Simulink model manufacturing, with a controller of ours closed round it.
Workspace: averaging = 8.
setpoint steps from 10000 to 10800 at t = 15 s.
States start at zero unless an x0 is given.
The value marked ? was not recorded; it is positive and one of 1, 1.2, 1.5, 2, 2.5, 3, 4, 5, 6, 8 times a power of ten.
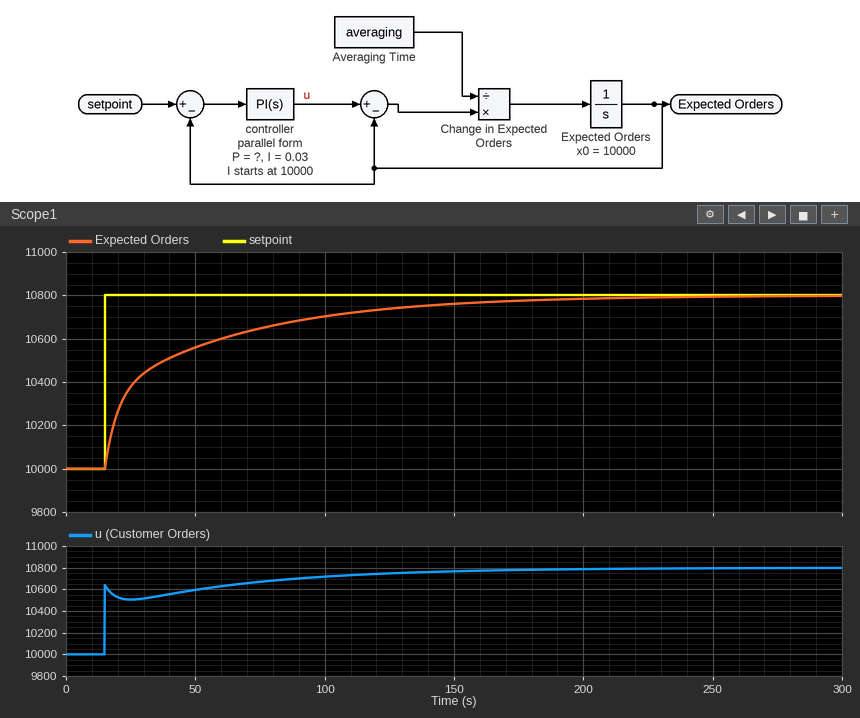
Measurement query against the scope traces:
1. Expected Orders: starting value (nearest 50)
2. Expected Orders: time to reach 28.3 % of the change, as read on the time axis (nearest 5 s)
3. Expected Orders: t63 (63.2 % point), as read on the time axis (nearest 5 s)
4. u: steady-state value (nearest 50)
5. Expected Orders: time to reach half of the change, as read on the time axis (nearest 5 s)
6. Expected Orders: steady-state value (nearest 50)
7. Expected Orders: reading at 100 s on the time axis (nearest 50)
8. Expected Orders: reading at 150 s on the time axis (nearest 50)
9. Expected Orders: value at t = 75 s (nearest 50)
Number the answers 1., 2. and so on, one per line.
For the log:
1. 10000
2. 20 s
3. 40 s
4. 10800
5. 25 s
6. 10800
7. 10700
8. 10750
9. 10650
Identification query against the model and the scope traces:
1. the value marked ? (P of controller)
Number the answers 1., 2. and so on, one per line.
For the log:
1. 0.8
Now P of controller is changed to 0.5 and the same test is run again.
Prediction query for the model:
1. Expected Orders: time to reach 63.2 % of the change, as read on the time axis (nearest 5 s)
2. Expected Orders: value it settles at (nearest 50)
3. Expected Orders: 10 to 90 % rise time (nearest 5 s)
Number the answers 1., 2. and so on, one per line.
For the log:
1. 45 s
2. 10800
3. 85 s
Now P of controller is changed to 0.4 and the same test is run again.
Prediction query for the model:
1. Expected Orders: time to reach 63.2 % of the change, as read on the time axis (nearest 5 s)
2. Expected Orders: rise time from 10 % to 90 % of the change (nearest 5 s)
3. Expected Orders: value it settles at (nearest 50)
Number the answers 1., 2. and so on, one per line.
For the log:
1. 45 s
2. 80 s
3. 10800
